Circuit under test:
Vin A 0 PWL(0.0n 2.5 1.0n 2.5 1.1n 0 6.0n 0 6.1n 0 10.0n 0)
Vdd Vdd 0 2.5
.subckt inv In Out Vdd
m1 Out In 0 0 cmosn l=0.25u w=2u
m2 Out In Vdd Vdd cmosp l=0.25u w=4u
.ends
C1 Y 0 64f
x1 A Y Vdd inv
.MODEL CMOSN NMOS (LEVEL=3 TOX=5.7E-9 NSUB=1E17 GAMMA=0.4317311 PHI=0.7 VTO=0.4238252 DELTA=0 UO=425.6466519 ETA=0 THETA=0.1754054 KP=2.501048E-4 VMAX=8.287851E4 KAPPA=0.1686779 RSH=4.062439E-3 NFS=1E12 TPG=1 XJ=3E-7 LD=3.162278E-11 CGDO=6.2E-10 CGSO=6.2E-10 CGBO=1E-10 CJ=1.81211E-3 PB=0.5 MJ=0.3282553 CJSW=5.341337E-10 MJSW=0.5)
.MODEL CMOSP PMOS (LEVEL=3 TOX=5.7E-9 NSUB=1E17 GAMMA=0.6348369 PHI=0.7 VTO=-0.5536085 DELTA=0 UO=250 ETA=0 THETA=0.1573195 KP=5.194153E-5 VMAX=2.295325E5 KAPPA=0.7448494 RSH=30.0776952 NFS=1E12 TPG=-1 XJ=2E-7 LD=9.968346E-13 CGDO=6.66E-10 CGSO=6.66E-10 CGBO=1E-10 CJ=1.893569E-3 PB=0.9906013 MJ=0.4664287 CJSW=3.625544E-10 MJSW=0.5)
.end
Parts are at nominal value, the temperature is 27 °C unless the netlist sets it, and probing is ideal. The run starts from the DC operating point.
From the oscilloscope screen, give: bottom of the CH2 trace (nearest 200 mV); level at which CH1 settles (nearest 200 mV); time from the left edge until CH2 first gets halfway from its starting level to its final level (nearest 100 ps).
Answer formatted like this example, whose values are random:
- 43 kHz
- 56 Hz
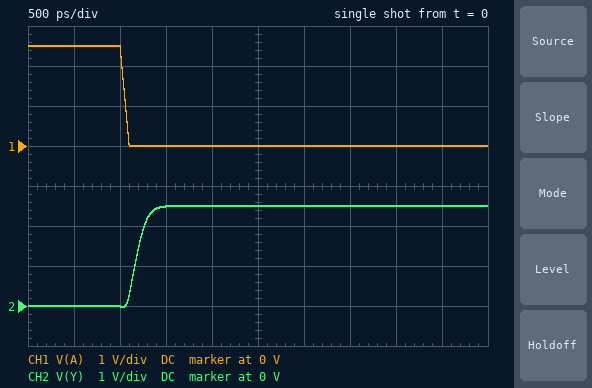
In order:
- 0 V
- 0 V
- 1.2 ns
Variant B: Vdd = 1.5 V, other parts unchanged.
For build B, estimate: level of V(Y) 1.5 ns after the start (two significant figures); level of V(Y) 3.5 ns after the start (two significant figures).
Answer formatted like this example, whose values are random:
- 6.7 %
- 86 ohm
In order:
- 1.4 V
- 1.5 V
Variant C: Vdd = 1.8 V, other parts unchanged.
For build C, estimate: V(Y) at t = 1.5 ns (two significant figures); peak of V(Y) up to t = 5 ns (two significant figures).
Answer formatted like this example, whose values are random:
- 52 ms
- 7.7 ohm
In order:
- 1.7 V
- 1.8 V
